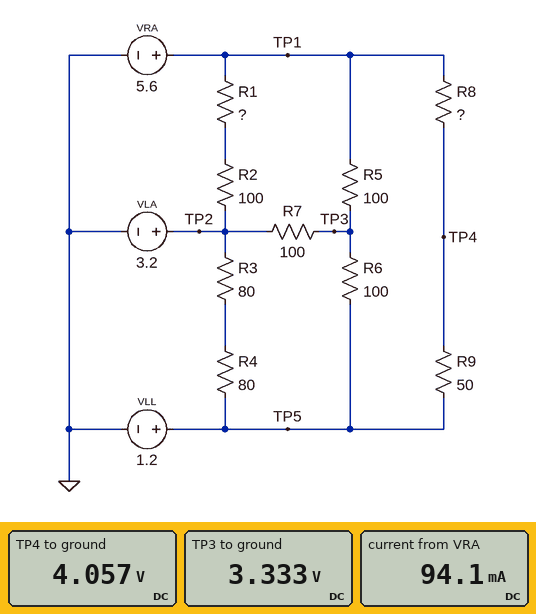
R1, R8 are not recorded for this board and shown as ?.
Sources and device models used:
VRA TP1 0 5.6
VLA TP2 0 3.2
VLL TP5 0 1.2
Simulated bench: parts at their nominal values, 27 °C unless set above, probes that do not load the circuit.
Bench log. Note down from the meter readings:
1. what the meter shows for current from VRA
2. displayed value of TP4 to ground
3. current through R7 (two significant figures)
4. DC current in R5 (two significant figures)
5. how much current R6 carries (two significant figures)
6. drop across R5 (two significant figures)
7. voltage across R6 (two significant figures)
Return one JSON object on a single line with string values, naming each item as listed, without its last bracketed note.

{"what the meter shows for current from VRA": "94.1 mA", "displayed value of TP4 to ground": "4.057 V", "current through R7": "1.3 mA", "DC current in R5": "23 mA", "how much current R6 carries": "21 mA", "drop across R5": "2.3 V", "voltage across R6": "2.1 V"}
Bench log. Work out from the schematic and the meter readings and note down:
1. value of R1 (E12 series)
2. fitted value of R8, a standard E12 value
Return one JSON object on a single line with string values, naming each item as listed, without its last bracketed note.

{"value of R1": "68 Ω", "fitted value of R8, a standard E12 value": "27 Ω"}
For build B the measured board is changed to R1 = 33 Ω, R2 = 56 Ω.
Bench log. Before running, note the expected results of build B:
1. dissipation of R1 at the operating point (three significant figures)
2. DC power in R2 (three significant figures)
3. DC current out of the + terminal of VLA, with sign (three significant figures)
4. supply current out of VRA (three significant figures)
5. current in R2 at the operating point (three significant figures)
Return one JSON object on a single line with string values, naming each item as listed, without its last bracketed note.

{"dissipation of R1 at the operating point": "24.0 mW", "DC power in R2": "40.7 mW", "DC current out of the + terminal of VLA, with sign": "-15.8 mA", "supply current out of VRA": "107 mA", "current in R2 at the operating point": "27.0 mA"}
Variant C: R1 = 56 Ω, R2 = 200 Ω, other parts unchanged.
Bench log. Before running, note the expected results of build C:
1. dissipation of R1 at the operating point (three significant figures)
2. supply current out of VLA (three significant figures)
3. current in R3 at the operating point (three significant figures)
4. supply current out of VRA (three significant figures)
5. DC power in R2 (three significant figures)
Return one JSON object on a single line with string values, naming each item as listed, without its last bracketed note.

{"dissipation of R1 at the operating point": "4.92 mW", "supply current out of VLA": "1.79 mA", "current in R3 at the operating point": "12.5 mA", "supply current out of VRA": "89.2 mA", "DC power in R2": "17.6 mW"}
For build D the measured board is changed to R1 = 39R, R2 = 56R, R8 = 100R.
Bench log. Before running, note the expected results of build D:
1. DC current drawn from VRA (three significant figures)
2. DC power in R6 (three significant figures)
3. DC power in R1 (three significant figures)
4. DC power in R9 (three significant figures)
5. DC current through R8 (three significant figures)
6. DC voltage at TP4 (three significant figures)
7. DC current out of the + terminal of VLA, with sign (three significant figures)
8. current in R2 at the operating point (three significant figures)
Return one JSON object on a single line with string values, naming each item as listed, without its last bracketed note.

{"DC current drawn from VRA": "77.3 mA", "DC power in R6": "45.5 mW", "DC power in R1": "24.9 mW", "DC power in R9": "43.0 mW", "DC current through R8": "29.3 mA", "DC voltage at TP4": "2.67 V", "DC current out of the + terminal of VLA, with sign": "-14.1 mA", "current in R2 at the operating point": "25.3 mA"}
